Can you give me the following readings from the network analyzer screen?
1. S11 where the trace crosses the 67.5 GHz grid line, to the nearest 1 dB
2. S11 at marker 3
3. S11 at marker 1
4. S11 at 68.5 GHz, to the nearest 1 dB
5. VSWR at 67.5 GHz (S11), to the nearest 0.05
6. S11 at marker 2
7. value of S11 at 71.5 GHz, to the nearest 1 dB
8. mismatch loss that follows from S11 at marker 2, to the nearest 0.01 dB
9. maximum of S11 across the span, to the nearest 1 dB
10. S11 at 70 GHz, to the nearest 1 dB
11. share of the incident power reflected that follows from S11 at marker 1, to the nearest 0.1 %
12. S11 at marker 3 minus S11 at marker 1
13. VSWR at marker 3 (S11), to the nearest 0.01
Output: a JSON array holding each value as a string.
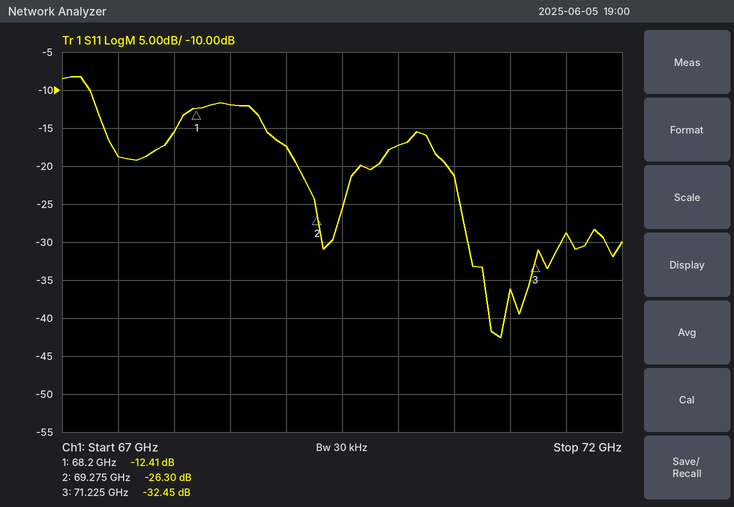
["-19 dB", "-32.45 dB", "-12.41 dB", "-12 dB", "1.25", "-26.30 dB", "-29 dB", "0.01 dB", "-8 dB", "-17 dB", "5.7 %", "-20.04 dB", "1.05"]
